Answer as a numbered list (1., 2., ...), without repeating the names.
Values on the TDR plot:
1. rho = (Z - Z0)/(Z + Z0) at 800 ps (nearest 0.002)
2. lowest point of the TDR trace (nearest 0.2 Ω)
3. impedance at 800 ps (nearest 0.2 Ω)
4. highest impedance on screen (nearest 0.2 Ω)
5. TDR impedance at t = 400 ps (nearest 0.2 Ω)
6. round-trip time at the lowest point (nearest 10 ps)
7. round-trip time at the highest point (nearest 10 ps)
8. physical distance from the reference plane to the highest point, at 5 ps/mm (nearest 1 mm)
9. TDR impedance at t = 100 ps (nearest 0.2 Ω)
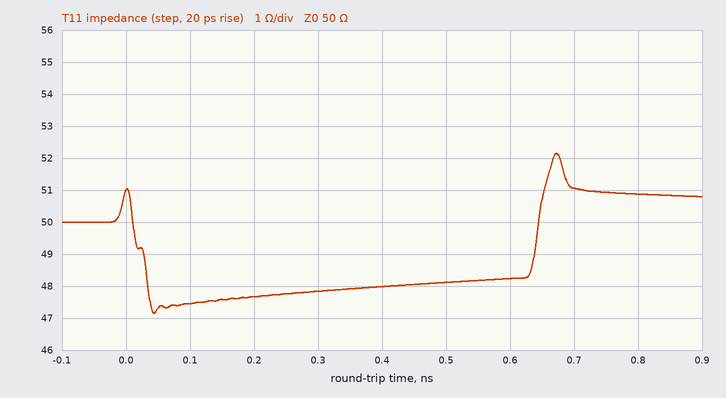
1. +0.008
2. 47.2 Ω
3. 50.8 Ω
4. 52.2 Ω
5. 48.0 Ω
6. 40 ps
7. 670 ps
8. 67 mm
9. 47.4 Ω
